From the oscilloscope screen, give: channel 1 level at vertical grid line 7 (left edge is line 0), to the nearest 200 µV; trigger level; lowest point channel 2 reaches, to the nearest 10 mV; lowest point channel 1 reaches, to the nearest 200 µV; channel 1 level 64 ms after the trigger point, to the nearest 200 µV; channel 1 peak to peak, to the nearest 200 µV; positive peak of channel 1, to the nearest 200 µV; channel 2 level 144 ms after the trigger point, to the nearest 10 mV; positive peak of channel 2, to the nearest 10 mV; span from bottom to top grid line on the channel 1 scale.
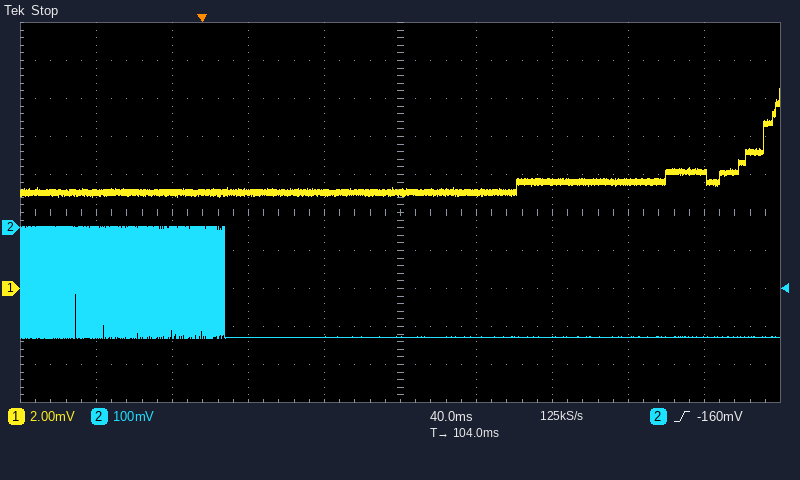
5.6 mV
-160 mV
-290 mV
4.8 mV
5.0 mV
5.8 mV
10.6 mV
-290 mV
0 mV
20 mV
